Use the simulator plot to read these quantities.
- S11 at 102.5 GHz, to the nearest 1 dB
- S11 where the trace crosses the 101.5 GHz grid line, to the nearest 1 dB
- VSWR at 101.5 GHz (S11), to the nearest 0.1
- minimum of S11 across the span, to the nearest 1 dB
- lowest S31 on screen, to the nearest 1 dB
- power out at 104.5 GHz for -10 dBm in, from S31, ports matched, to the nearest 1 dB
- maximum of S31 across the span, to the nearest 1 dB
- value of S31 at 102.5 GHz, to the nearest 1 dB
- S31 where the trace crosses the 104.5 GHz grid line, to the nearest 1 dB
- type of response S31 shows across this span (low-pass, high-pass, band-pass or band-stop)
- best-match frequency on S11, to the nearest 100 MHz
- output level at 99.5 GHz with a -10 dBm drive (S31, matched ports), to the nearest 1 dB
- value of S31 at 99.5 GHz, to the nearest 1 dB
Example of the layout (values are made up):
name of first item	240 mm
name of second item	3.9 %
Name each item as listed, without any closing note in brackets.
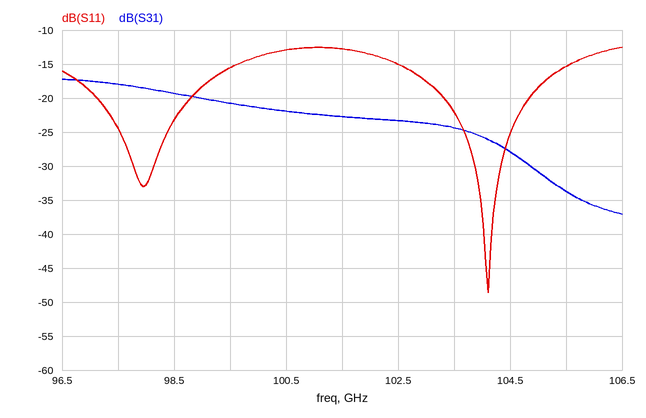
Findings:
S11 at 102.5 GHz, to the nearest 1 dB	-15 dB
S11 where the trace crosses the 101.5 GHz grid line, to the nearest 1 dB	-13 dB
VSWR at 101.5 GHz (S11), to the nearest 0.1	1.6
minimum of S11 across the span, to the nearest 1 dB	-49 dB
lowest S31 on screen, to the nearest 1 dB	-37 dB
power out at 104.5 GHz for -10 dBm in, from S31, ports matched, to the nearest 1 dB	-38 dBm
maximum of S31 across the span, to the nearest 1 dB	-17 dB
value of S31 at 102.5 GHz, to the nearest 1 dB	-23 dB
S31 where the trace crosses the 104.5 GHz grid line, to the nearest 1 dB	-28 dB
type of response S31 shows across this span	low-pass
best-match frequency on S11, to the nearest 100 MHz	104.1 GHz
output level at 99.5 GHz with a -10 dBm drive (S31, matched ports), to the nearest 1 dB	-31 dBm
value of S31 at 99.5 GHz, to the nearest 1 dB	-21 dB
